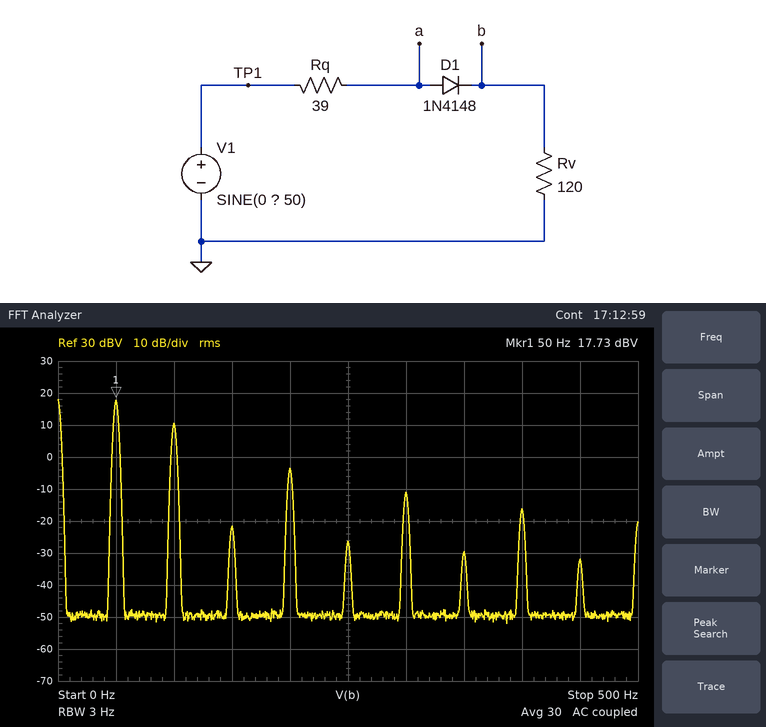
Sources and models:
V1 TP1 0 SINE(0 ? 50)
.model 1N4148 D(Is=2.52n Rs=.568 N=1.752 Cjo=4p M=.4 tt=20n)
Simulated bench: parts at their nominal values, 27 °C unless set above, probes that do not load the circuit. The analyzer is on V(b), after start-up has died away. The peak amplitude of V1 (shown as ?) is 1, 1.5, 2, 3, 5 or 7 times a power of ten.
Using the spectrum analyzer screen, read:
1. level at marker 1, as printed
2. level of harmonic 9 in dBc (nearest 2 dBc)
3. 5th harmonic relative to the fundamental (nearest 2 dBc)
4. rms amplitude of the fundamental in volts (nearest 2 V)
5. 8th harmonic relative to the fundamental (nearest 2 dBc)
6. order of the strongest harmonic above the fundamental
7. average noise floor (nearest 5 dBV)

17.73 dBV
-50 dBc
-44 dBc
8 V
-34 dBc
2
-50 dBV
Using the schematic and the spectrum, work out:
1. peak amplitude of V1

30 V
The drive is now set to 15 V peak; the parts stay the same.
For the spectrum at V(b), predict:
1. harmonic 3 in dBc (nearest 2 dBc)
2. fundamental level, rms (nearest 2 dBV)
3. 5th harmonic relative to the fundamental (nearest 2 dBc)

-34 dBc
12 dBV
-38 dBc
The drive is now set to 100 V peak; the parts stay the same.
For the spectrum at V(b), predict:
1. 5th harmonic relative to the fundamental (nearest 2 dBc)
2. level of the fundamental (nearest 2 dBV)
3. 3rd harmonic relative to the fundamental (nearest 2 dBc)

-54 dBc
28 dBV
-50 dBc
